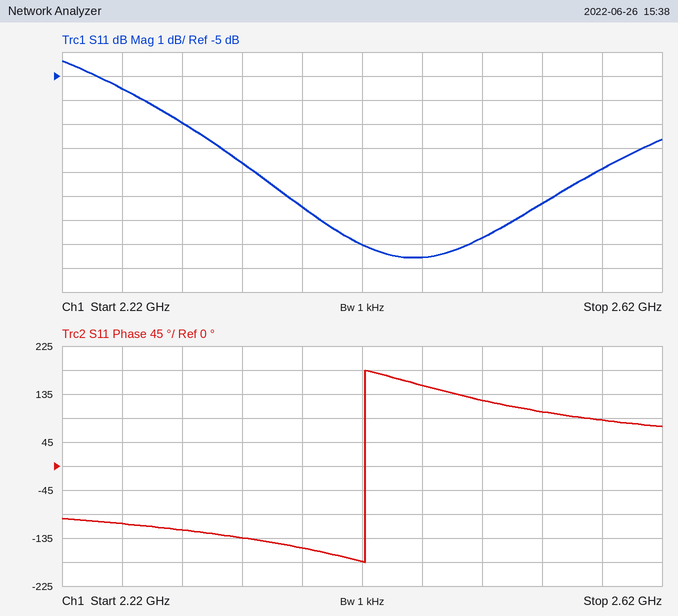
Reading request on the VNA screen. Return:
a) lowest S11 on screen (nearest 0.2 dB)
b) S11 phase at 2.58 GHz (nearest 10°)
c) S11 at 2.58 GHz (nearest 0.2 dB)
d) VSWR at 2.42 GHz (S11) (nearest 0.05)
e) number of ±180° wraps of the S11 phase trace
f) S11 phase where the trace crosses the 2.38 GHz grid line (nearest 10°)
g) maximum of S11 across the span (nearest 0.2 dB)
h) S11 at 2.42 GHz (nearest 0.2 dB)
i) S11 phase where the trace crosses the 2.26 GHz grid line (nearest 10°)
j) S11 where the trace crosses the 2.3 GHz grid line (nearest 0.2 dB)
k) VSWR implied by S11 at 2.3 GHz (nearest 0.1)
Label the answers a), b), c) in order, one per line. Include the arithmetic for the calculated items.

a) -12.6 dB
b) 90°
c) -8.8 dB
d) |Γ| = 10^(-12/20) = 0.2512; VSWR = (1 + 0.2512)/(1 − 0.2512) ≈ 1.67, so 1.65 to the nearest 0.05
e) 1
f) -150°
g) -4.4 dB
h) -12.0 dB
i) -110°
j) -7.0 dB
k) |Γ| = 10^(-7/20) = 0.4467; VSWR = (1 + 0.4467)/(1 − 0.4467) ≈ 2.6
